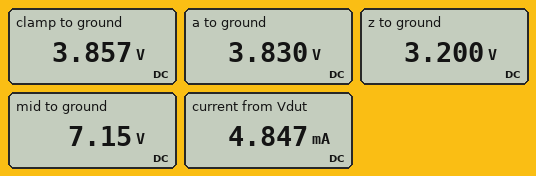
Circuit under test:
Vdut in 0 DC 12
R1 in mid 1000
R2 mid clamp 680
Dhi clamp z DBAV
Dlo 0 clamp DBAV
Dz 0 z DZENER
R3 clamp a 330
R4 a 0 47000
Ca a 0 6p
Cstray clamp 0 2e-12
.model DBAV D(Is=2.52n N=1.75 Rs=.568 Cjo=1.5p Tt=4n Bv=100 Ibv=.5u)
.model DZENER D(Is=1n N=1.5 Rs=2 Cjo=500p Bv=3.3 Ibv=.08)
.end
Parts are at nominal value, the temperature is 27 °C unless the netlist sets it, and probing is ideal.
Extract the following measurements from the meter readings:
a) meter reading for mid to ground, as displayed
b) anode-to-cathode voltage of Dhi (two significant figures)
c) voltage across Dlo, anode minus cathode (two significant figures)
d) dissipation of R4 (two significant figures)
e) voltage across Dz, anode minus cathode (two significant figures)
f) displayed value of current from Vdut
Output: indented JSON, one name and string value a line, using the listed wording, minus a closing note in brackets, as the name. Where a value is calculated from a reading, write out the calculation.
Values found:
{
  "meter reading for mid to ground, as displayed": "7.15 V",
  "anode-to-cathode voltage of Dhi": "3.857 V - 3.2 V = 660 mV",
  "voltage across Dlo, anode minus cathode": "0 V - 3.857 V = -3.9 V",
  "dissipation of R4": "(3.83 V)^2 / 47 kΩ = 310 µW",
  "voltage across Dz, anode minus cathode": "0 V - 3.2 V = -3.2 V",
  "displayed value of current from Vdut": "4.847 mA"
}
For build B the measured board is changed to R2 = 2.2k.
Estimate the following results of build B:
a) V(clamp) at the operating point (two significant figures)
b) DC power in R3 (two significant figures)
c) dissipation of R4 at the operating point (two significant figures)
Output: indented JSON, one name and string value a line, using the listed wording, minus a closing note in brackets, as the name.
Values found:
{
  "V(clamp) at the operating point": "3.8 V",
  "DC power in R3": "2.1 µW",
  "dissipation of R4 at the operating point": "300 µW"
}
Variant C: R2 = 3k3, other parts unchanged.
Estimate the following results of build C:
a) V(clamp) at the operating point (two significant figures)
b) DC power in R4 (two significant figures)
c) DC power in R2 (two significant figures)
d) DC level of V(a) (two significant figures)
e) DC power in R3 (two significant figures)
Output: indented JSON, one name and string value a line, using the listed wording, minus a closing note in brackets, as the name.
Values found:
{
  "V(clamp) at the operating point": "3.8 V",
  "DC power in R4": "300 µW",
  "DC power in R2": "12 mW",
  "DC level of V(a)": "3.7 V",
  "DC power in R3": "2.1 µW"
}
